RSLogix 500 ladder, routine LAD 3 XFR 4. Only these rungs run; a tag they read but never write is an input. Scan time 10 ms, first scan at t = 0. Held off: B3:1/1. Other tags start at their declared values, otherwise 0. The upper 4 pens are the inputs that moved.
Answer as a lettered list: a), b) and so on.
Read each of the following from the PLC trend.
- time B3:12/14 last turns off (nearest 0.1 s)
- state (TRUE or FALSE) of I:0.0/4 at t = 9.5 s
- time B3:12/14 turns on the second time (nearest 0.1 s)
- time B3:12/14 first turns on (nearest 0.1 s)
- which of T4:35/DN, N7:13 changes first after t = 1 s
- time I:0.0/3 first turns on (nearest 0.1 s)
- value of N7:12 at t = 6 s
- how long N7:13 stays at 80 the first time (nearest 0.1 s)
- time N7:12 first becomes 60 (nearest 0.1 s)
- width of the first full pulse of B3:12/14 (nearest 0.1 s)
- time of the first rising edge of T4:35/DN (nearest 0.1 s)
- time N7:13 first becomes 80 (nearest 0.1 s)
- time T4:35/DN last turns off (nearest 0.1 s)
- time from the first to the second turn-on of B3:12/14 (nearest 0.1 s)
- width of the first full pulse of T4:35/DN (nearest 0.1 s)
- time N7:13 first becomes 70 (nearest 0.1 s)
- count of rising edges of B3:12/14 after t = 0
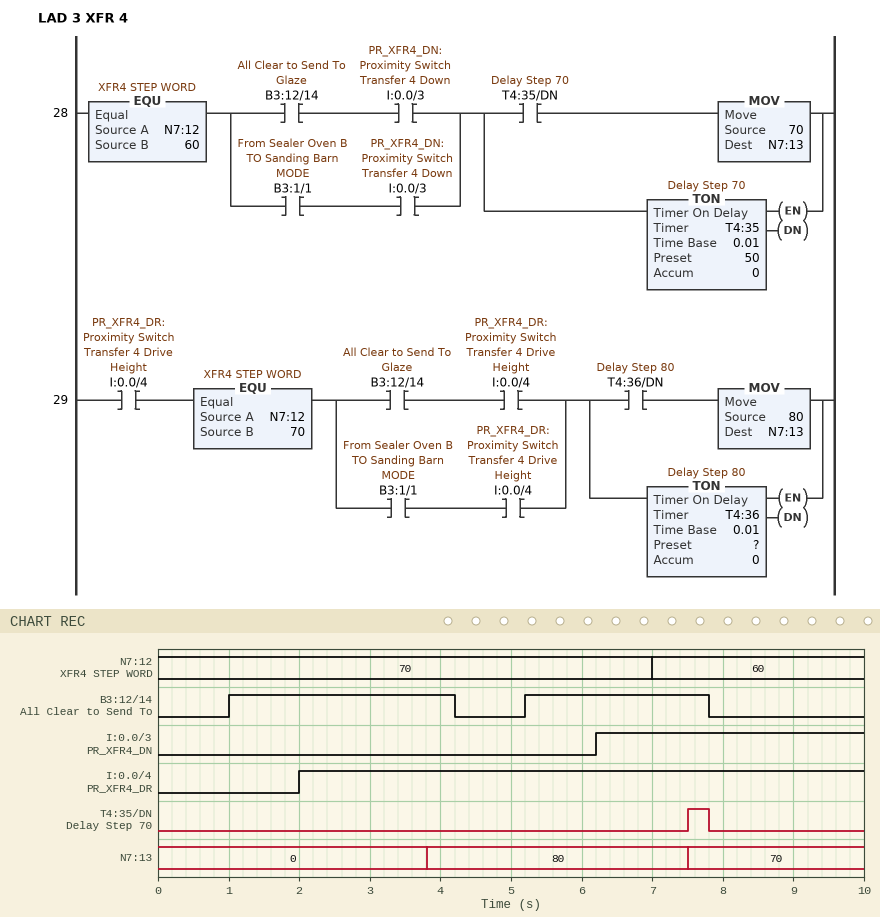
a) 7.8 s
b) TRUE
c) 5.2 s
d) 1.0 s
e) N7:13
f) 6.2 s
g) 70
h) 3.7 s
i) 7.0 s
j) 3.2 s
k) 7.5 s
l) 3.8 s
m) 7.8 s
n) 4.2 s
o) 0.3 s
p) 7.5 s
q) 2
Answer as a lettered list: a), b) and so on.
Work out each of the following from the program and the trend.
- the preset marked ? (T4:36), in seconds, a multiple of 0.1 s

a) 1.8 s
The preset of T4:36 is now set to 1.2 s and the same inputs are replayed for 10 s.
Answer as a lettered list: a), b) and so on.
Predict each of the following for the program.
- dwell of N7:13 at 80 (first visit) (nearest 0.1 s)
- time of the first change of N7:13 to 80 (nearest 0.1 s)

a) 4.3 s
b) 3.2 s
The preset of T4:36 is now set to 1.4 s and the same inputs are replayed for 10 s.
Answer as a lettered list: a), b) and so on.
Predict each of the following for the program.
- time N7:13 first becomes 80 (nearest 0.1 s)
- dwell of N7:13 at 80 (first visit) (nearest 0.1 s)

a) 3.4 s
b) 4.1 s
